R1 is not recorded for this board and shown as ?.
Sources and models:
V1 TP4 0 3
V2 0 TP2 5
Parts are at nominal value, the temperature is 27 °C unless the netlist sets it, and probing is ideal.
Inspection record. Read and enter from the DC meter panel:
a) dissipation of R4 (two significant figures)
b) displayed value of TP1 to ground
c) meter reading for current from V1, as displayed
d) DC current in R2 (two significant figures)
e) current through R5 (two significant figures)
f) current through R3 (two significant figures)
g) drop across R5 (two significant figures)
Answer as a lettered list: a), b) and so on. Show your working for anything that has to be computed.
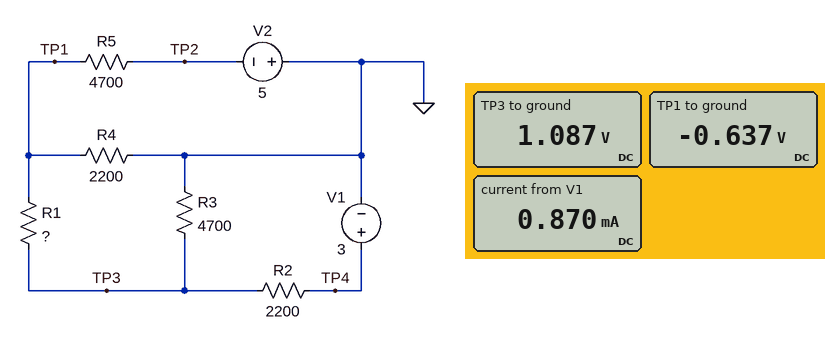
a) (0 V - (-637 mV))^2 / 2.2 kΩ = 180 µW
b) -0.637 V
c) 0.870 mA
d) (3 V - 1.087 V) / 2.2 kΩ = 870 µA
e) (-637 mV - (-5 V)) / 4.7 kΩ = 930 µA
f) (1.087 V) / 4.7 kΩ = 230 µA
g) -637 mV - (-5 V) = 4.4 V
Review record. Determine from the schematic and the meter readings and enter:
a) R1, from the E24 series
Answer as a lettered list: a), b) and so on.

a) 2.7 kΩ
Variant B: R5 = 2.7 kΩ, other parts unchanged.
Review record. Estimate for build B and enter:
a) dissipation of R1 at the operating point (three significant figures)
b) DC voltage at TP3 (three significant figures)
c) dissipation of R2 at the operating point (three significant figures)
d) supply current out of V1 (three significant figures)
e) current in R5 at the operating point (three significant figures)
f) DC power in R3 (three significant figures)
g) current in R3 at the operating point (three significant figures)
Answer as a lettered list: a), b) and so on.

a) 1.70 mW
b) 856 mV
c) 2.09 mW
d) 975 µA
e) 1.38 mA
f) 156 µW
g) 182 µA
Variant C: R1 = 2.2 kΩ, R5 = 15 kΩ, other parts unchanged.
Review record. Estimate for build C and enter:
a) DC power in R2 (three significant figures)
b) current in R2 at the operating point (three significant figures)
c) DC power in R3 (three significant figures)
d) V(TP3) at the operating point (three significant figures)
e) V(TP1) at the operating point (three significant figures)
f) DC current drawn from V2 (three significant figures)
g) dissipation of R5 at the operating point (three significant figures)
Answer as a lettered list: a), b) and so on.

a) 1.27 mW
b) 760 µA
c) 375 µW
d) 1.33 V
e) 277 mV
f) 352 µA
g) 1.86 mW
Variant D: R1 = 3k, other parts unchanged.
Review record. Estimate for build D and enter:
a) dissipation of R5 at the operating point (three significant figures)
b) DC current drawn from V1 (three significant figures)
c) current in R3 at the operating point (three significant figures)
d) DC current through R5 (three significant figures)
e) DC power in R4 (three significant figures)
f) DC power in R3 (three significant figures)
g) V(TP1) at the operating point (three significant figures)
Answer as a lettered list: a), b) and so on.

a) 3.96 mW
b) 848 µA
c) 241 µA
d) 918 µA
e) 213 µW
f) 274 µW
g) -685 mV
